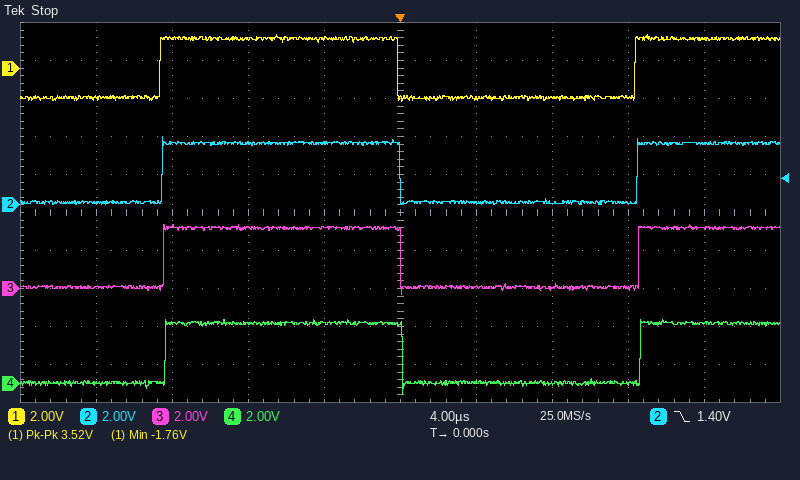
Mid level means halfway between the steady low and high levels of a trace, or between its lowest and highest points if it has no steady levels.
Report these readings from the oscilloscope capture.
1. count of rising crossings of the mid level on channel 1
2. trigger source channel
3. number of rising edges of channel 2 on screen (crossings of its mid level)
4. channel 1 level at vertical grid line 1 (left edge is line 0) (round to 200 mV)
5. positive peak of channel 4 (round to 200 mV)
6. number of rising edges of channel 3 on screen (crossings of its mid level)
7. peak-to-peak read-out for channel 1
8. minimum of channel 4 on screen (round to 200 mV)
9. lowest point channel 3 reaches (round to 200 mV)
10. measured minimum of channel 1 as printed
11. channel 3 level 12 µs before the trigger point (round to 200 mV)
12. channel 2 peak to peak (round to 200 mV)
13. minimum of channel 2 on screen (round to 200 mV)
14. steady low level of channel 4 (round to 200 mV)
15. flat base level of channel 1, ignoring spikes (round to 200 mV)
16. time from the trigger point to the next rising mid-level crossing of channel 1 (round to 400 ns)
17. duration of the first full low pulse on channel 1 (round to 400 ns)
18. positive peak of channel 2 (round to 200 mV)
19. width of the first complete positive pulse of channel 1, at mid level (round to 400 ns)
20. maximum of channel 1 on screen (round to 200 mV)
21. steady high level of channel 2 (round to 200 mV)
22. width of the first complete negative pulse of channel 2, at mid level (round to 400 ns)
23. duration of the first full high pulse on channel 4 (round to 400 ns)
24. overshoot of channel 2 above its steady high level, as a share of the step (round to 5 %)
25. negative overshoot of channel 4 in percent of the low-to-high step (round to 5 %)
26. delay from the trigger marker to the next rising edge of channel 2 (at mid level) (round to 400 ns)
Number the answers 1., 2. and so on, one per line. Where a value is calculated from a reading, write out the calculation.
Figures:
1. 2
2. channel 2
3. 2
4. -1.6 V
5. 3.4 V
6. 2
7. 3.52 V
8. -600 mV
9. -400 mV
10. -1.76 V
11. 3.2 V
12. 3.6 V − (0.0 V) = 3.6 V
13. 0.0 V
14. 0.0 V
15. -1.6 V
16. 12.4 µs
17. 12.4 µs
18. 3.6 V
19. 12.4 µs
20. 1.8 V
21. 3.2 V
22. 12.4 µs
23. 12.4 µs
24. 10 %
25. 20 %
26. 12.4 µs
